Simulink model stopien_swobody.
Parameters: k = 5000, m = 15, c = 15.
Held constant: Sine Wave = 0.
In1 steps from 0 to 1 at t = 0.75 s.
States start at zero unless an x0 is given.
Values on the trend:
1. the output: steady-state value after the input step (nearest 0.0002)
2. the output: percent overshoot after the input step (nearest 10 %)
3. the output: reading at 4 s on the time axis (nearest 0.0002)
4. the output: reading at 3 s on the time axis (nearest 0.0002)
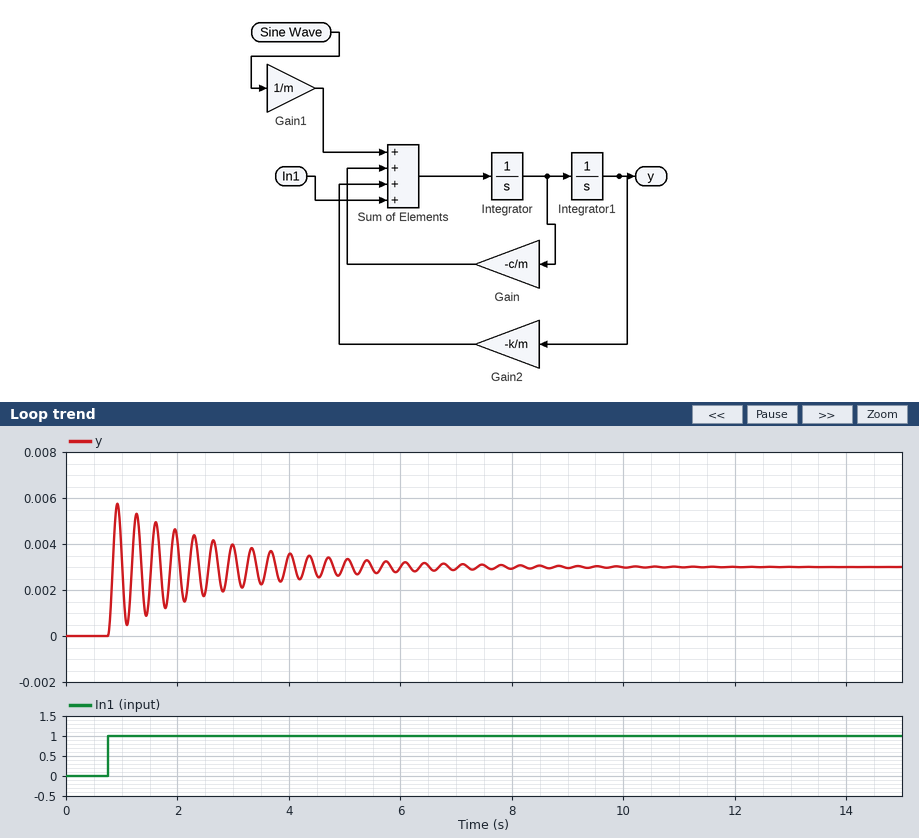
0.0030
90 %
0.0036
0.0040
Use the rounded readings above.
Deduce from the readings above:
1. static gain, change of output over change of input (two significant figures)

0.0030
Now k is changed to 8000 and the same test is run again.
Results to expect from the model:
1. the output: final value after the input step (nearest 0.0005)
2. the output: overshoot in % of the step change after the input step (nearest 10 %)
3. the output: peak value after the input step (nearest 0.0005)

0.0020
90 %
0.0035
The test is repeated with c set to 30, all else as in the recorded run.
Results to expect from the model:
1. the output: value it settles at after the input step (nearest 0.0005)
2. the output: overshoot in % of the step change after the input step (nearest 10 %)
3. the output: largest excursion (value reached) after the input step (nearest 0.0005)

0.0030
80 %
0.0055
